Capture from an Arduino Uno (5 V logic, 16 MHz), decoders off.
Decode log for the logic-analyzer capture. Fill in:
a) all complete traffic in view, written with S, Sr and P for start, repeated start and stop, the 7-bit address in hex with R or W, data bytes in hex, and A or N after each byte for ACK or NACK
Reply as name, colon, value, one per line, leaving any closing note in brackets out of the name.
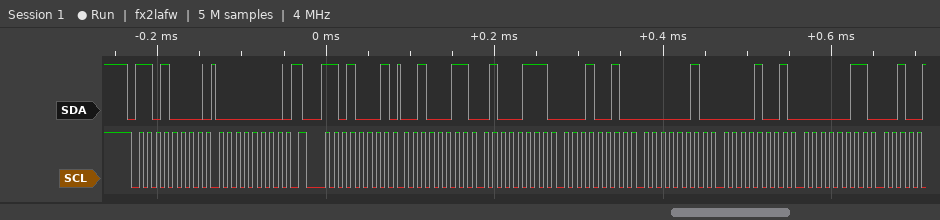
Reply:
all complete traffic in view, written with S, Sr and P for start, repeated start and stop, the 7-bit address in hex with R or W, data bytes in hex, and A or N after each byte for ACK or NACK: S 68W A 00 A Sr 68R A 23 A 47 A 12 A 02 A 09 A 03 A
